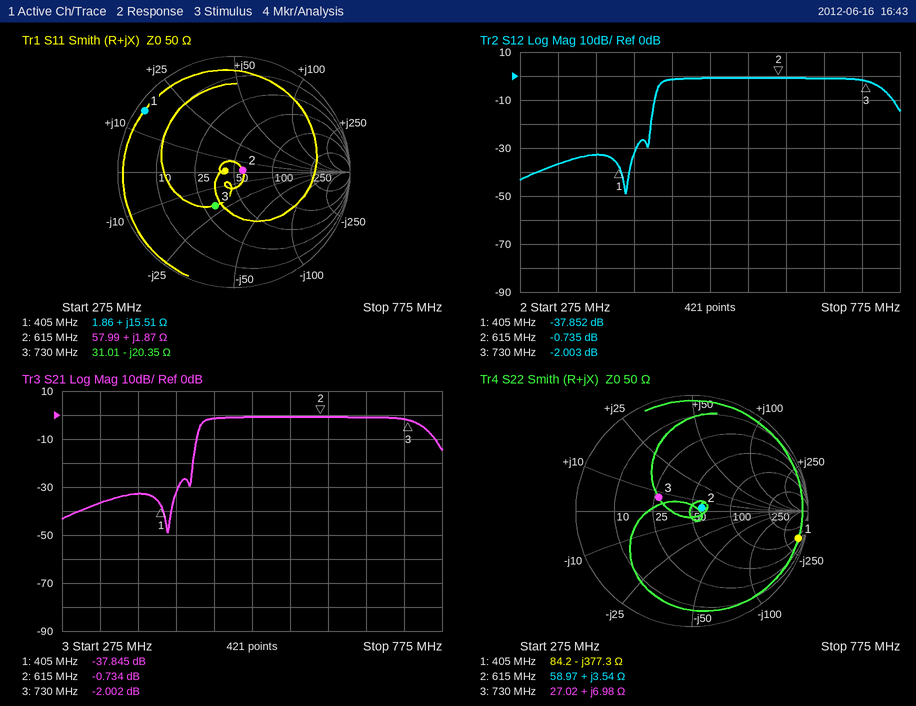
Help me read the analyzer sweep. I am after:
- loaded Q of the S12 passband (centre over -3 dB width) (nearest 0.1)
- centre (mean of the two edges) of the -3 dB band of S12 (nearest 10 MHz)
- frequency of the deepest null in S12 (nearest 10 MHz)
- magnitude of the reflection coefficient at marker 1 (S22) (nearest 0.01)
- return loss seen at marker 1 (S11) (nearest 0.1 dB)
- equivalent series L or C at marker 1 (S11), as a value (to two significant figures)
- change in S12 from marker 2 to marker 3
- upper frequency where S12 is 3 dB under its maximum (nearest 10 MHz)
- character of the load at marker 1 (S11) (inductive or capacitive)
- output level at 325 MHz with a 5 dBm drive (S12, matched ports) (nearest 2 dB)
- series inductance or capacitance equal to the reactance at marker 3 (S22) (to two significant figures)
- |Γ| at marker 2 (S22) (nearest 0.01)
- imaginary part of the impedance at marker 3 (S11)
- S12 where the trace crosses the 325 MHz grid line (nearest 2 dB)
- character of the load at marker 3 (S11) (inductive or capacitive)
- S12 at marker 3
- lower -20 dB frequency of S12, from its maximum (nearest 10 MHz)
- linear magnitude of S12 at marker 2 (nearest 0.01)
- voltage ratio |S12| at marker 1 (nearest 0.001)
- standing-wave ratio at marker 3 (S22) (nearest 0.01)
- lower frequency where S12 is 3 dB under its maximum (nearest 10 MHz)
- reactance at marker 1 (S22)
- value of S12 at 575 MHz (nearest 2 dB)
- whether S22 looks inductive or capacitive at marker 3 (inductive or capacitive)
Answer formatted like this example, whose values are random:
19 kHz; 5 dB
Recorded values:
2.1; 600 MHz; 410 MHz; 0.95; 0.6 dB; 6.1 nH; -1.268 dB; 740 MHz; inductive; -32 dBm; 1.5 nH; 0.09; -20.35 Ω; -36 dB; capacitive; -2.003 dB; 450 MHz; 0.92; 0.013; 1.90; 460 MHz; -377.3 Ω; 0 dB; inductive
